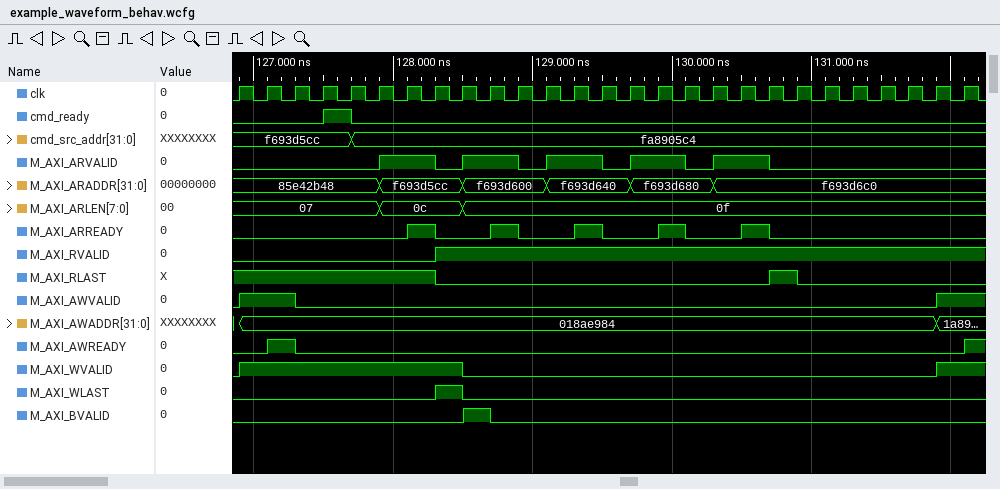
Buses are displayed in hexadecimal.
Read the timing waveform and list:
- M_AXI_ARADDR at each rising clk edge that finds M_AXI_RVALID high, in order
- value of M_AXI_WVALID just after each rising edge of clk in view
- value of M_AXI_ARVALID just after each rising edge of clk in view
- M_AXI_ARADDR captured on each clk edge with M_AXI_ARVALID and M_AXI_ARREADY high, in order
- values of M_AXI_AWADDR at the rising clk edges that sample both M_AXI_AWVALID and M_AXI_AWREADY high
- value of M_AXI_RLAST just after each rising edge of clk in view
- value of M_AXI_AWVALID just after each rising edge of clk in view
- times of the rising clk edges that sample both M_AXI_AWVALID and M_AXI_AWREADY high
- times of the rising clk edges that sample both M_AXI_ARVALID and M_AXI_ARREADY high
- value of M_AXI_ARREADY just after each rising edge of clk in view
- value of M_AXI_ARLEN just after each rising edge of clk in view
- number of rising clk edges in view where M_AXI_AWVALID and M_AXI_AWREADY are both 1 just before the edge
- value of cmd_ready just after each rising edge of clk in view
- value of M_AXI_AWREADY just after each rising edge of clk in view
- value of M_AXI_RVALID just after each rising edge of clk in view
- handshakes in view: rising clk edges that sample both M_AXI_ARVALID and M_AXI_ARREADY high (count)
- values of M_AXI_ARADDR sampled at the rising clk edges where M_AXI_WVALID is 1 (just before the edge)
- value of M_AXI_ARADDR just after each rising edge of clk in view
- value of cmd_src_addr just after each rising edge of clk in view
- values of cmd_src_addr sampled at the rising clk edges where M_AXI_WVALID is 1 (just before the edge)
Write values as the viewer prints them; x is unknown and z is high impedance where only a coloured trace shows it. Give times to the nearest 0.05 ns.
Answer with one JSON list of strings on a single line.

["f693d5cc, f693d600, f693d600, f693d600, f693d640, f693d640, f693d640, f693d680, f693d680, f693d680, f693d6c0, f693d6c0, f693d6c0, f693d6c0, f693d6c0, f693d6c0, f693d6c0, f693d6c0, f693d6c0", "1 1 1 1 1 1 1 1 0 0 0 0 0 0 0 0 0 0 0 0 0 0 0 0 0 1 1", "0 0 0 0 0 1 1 0 1 1 0 1 1 0 1 1 0 1 1 0 0 0 0 0 0 0 0", "f693d5cc, f693d600, f693d640, f693d680, f693d6c0", "018ae984", "1 1 1 1 1 1 1 0 0 0 0 0 0 0 0 0 0 0 0 1 0 0 0 0 0 0 0", "1 1 0 0 0 0 0 0 0 0 0 0 0 0 0 0 0 0 0 0 0 0 0 0 0 1 1", "127.3 ns", "128.3 ns, 128.9 ns, 129.5 ns, 130.1 ns, 130.7 ns", "0 0 0 0 0 0 1 0 0 1 0 0 1 0 0 1 0 0 1 0 0 0 0 0 0 0 0", "07, 07, 07, 07, 07, 0c, 0c, 0c, 0f, 0f, 0f, 0f, 0f, 0f, 0f, 0f, 0f, 0f, 0f, 0f, 0f, 0f, 0f, 0f, 0f, 0f, 0f", "1", "0 0 0 1 0 0 0 0 0 0 0 0 0 0 0 0 0 0 0 0 0 0 0 0 0 0 0", "0 1 0 0 0 0 0 0 0 0 0 0 0 0 0 0 0 0 0 0 0 0 0 0 0 0 1", "0 0 0 0 0 0 0 1 1 1 1 1 1 1 1 1 1 1 1 1 1 1 1 1 1 1 1", "5", "85e42b48, 85e42b48, 85e42b48, 85e42b48, 85e42b48, f693d5cc, f693d5cc, f693d5cc, f693d6c0", "85e42b48, 85e42b48, 85e42b48, 85e42b48, 85e42b48, f693d5cc, f693d5cc, f693d5cc, f693d600, f693d600, f693d600, f693d640, f693d640, f693d640, f693d680, f693d680, f693d680, f693d6c0, f693d6c0, f693d6c0, f693d6c0, f693d6c0, f693d6c0, f693d6c0, f693d6c0, f693d6c0, f693d6c0", "f693d5cc, f693d5cc, f693d5cc, f693d5cc, fa8905c4, fa8905c4, fa8905c4, fa8905c4, fa8905c4, fa8905c4, fa8905c4, fa8905c4, fa8905c4, fa8905c4, fa8905c4, fa8905c4, fa8905c4, fa8905c4, fa8905c4, fa8905c4, fa8905c4, fa8905c4, fa8905c4, fa8905c4, fa8905c4, fa8905c4, fa8905c4", "f693d5cc, f693d5cc, f693d5cc, f693d5cc, fa8905c4, fa8905c4, fa8905c4, fa8905c4, fa8905c4"]
